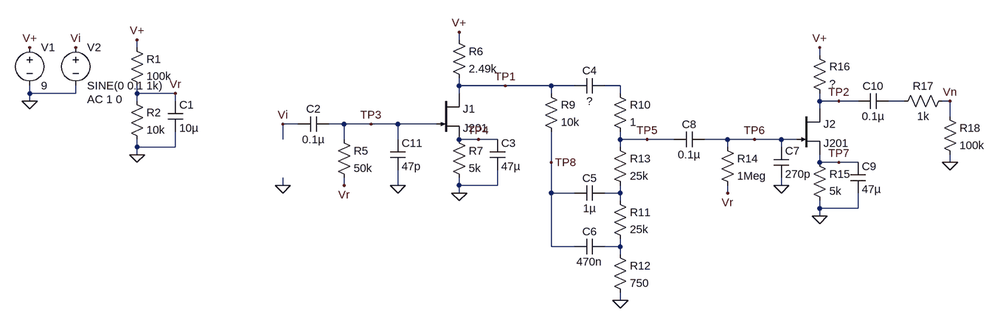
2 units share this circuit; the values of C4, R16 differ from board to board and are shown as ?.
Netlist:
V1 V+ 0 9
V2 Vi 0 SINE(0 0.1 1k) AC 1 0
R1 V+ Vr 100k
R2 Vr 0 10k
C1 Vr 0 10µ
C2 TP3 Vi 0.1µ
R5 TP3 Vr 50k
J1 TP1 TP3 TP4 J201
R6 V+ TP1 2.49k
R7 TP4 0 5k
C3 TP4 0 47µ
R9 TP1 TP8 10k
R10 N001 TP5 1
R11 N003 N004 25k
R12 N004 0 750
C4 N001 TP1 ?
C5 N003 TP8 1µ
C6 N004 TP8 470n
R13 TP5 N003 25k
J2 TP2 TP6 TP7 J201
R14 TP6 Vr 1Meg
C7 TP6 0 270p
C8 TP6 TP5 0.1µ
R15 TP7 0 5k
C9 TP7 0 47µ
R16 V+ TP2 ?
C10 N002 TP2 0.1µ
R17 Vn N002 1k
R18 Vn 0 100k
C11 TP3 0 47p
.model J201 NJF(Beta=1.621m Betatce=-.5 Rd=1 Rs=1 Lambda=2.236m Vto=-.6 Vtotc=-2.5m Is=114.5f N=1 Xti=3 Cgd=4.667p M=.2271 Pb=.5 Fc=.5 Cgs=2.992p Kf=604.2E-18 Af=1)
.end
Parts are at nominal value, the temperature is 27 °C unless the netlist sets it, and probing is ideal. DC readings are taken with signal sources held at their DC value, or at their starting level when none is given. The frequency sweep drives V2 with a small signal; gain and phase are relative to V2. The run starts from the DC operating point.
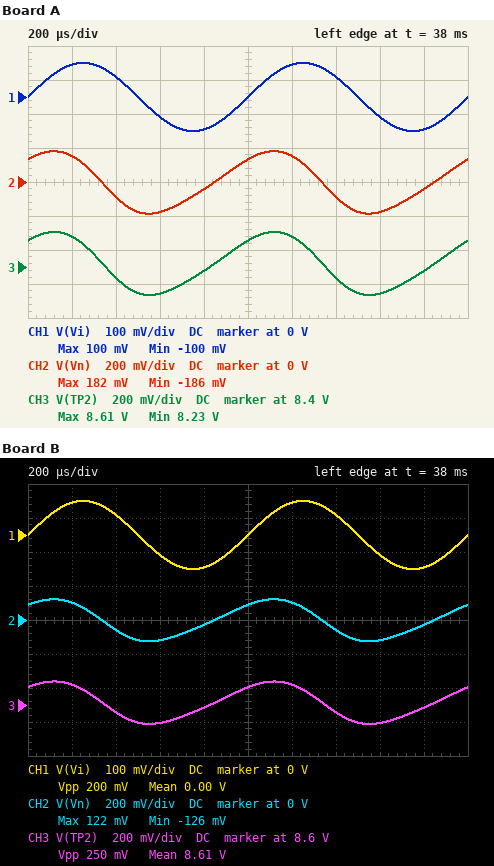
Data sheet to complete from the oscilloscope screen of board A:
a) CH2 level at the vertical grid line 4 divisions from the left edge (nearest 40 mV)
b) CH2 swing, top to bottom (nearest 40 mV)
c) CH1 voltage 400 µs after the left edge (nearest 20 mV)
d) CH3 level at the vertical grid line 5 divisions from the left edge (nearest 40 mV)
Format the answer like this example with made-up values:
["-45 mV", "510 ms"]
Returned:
["-40 mV", "360 mV", "60 mV", "8.56 V"]
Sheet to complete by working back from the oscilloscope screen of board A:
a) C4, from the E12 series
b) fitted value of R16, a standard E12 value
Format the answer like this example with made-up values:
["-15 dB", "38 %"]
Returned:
["1.8 nF", "2.7 kΩ"]
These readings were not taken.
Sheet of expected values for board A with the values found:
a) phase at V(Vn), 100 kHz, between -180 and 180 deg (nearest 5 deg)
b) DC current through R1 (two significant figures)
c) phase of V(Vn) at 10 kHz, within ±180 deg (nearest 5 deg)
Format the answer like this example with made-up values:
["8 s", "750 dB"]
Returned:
["-15 deg", "82 µA", "15 deg"]
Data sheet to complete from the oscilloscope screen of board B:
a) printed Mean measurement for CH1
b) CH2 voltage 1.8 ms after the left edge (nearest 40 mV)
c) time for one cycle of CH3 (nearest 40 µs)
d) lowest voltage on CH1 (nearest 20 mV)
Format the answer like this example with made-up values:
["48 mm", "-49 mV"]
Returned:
["0.00 V", "-40 mV", "1.00 ms", "-100 mV"]
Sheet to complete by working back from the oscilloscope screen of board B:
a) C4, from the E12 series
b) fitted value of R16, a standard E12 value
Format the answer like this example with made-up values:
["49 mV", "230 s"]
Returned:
["1.8 nF", "1.8 kΩ"]
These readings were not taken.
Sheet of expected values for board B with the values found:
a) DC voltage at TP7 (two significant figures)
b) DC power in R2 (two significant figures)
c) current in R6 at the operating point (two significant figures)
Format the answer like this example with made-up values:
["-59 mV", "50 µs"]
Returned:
["1.1 V", "67 µW", "210 µA"]
